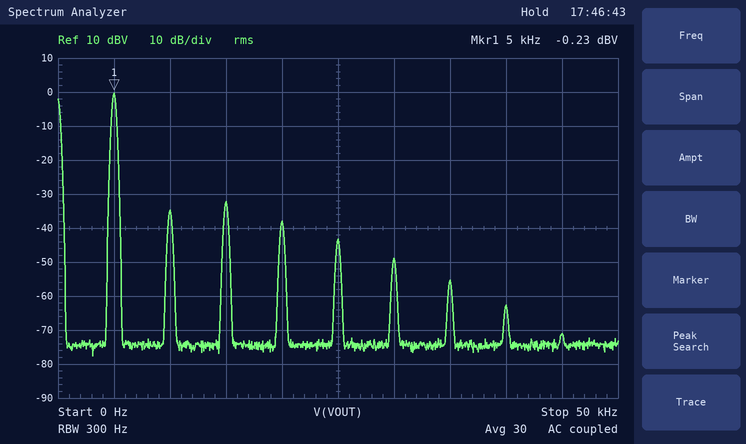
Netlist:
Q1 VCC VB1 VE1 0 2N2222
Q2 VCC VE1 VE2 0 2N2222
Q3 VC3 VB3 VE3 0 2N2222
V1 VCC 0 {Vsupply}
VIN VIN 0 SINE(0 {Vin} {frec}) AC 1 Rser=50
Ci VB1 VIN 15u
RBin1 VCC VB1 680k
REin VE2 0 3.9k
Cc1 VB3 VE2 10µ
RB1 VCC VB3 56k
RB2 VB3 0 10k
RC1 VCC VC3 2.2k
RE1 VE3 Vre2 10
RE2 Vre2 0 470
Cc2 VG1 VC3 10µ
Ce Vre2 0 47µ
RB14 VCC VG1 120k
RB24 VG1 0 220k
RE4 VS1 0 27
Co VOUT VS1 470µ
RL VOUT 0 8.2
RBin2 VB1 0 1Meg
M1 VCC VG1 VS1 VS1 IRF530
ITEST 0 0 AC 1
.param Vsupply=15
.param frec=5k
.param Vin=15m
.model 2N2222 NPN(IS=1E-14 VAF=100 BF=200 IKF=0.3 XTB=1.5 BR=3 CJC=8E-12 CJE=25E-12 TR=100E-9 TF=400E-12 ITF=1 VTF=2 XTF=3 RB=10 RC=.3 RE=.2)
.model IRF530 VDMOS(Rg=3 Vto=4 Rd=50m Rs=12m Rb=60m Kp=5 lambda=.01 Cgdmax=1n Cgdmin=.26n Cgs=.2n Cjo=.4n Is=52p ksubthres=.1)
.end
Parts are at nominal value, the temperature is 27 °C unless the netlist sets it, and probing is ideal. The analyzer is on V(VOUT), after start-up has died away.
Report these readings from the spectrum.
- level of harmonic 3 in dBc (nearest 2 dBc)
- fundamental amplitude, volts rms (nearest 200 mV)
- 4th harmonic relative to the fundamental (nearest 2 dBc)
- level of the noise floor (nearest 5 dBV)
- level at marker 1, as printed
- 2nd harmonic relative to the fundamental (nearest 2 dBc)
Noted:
-32 dBc
1.0 V
-38 dBc
-75 dBV
-0.23 dBV
-34 dBc
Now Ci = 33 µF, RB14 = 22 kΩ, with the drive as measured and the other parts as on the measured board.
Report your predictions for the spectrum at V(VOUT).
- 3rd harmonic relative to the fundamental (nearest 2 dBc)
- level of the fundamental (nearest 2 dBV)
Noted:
-50 dBc
0 dBV
